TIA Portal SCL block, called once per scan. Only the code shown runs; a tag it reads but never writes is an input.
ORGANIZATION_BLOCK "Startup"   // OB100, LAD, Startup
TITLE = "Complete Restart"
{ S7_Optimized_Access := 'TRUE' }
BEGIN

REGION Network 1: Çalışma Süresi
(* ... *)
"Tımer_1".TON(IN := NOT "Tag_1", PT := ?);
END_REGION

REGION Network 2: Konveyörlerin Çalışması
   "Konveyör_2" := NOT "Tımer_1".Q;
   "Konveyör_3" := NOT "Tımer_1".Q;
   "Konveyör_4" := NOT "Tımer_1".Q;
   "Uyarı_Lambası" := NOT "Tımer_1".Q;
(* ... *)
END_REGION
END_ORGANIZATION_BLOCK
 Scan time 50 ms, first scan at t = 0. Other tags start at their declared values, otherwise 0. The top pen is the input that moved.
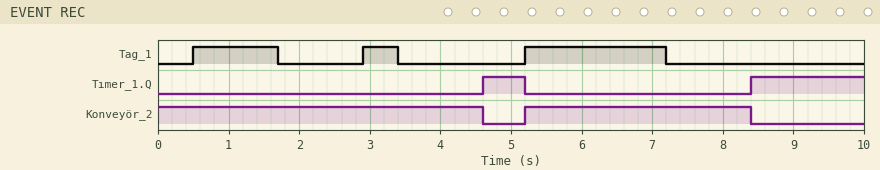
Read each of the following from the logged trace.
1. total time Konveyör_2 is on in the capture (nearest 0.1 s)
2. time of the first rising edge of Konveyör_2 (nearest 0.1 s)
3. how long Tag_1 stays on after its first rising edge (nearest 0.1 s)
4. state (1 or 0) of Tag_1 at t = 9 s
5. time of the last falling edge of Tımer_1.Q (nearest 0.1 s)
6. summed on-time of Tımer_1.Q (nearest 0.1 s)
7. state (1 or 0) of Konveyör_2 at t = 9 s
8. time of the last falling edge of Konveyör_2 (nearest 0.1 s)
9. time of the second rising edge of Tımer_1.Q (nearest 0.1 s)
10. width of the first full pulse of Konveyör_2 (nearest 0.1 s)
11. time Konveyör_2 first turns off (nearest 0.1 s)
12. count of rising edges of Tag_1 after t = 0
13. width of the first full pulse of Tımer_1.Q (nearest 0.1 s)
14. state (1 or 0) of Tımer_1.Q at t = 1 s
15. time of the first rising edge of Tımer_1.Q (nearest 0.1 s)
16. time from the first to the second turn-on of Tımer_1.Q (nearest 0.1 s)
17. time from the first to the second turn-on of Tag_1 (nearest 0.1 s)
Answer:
7.8 s
5.2 s
1.2 s
0
5.2 s
2.2 s
0
8.4 s
8.4 s
3.2 s
4.6 s
3
0.6 s
0
4.6 s
3.8 s
2.4 s
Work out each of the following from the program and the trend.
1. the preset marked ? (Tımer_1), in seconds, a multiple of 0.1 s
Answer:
1.2 s
